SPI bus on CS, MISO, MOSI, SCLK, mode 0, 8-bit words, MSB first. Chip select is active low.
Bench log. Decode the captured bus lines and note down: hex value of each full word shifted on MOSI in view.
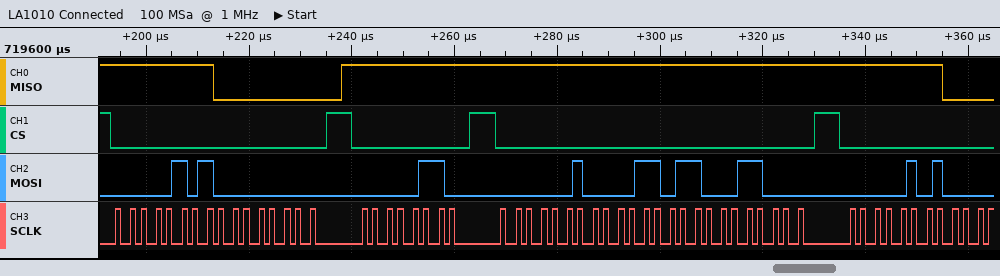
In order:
05, 00, 06, 02, 1B, 18, 05
